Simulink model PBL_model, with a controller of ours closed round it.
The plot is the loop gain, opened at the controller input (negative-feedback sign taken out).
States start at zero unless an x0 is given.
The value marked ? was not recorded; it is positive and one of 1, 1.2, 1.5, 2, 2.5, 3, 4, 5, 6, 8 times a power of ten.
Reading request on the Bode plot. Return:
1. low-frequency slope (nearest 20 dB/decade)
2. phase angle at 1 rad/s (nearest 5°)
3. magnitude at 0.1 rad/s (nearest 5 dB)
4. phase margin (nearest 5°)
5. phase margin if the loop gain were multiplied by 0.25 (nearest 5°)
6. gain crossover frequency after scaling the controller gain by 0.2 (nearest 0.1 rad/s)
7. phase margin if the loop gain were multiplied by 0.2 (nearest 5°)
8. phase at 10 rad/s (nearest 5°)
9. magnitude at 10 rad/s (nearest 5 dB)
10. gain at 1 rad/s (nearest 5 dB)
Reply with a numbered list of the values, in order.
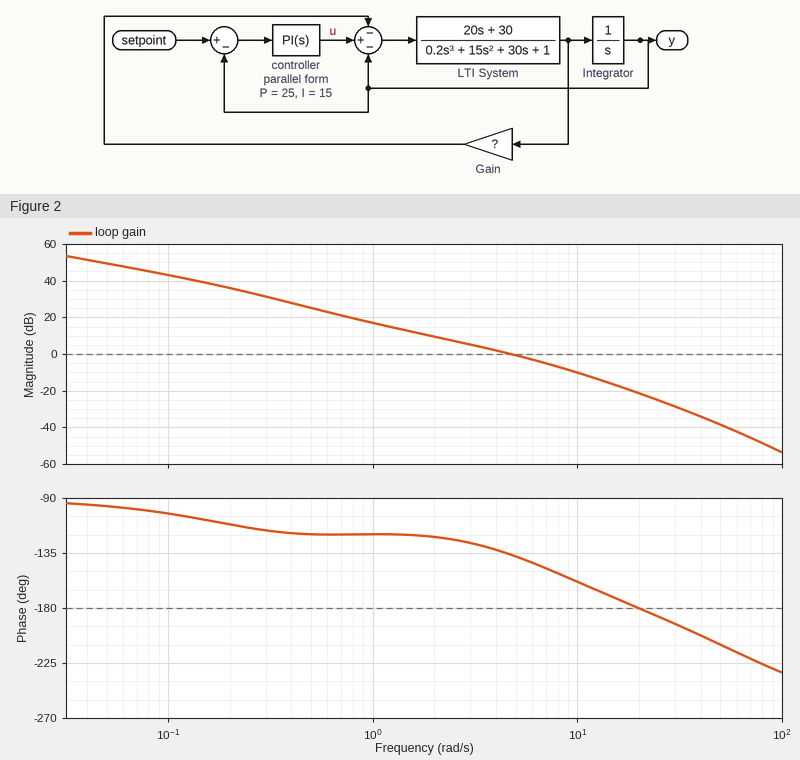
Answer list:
1. -20 dB/decade
2. -120°
3. 45 dB
4. 45°
5. 60°
6. 1.3 rad/s
7. 60°
8. -160°
9. -10 dB
10. 15 dB
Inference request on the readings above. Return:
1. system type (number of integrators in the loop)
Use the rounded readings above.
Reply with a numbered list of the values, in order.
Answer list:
1. 1
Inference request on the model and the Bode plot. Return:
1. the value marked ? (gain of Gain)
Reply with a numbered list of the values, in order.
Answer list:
1. 4
